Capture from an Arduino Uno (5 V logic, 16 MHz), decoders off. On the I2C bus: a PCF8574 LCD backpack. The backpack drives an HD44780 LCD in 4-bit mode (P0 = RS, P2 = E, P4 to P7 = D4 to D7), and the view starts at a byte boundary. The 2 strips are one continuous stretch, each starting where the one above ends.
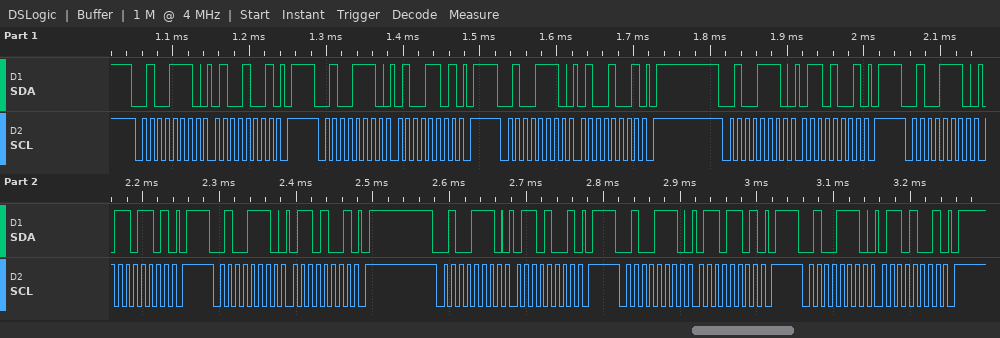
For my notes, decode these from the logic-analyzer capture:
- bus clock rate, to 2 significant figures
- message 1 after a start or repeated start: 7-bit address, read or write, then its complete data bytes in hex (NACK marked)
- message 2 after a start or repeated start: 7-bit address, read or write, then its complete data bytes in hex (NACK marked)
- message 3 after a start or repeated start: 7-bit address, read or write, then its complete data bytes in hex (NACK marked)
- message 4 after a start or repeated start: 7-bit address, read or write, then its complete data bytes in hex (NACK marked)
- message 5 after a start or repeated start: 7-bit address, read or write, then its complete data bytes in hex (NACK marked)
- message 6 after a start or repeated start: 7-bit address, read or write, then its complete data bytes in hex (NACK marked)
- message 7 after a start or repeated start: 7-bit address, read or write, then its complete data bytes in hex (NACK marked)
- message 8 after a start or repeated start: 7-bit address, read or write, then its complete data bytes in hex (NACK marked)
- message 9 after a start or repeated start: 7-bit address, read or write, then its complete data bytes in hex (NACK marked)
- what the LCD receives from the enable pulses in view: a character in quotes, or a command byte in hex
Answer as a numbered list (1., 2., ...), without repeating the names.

1. 100 kHz
2. 0x27 write: 49
3. 0x27 write: 4D
4. 0x27 write: 49
5. 0x27 write: 69
6. 0x27 write: 6D
7. 0x27 write: 69
8. 0x27 write: 69
9. 0x27 write: 6D
10. 0x27 write: 69
11. 'F'
